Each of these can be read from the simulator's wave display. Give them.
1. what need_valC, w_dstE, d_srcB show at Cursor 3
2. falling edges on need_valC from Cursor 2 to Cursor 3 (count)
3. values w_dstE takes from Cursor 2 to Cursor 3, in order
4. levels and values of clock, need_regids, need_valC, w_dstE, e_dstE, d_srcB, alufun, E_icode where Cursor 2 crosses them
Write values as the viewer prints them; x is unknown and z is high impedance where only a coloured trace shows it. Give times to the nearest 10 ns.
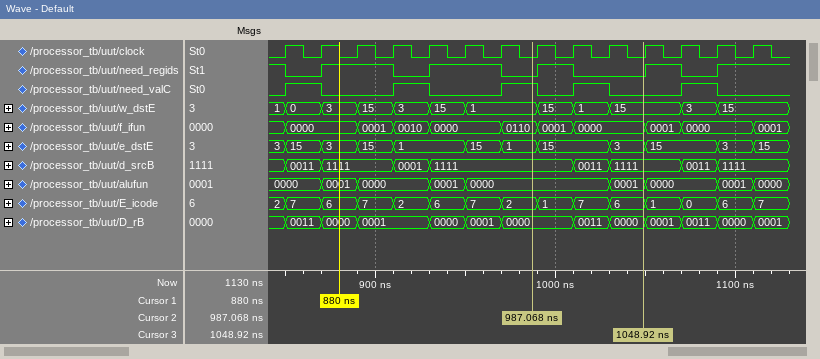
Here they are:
need_valC=0, w_dstE=15, d_srcB=1111
2
1, 15, 1, 15
clock=0, need_regids=0, need_valC=1, w_dstE=1, e_dstE=1, d_srcB=1111, alufun=0000, E_icode=2
